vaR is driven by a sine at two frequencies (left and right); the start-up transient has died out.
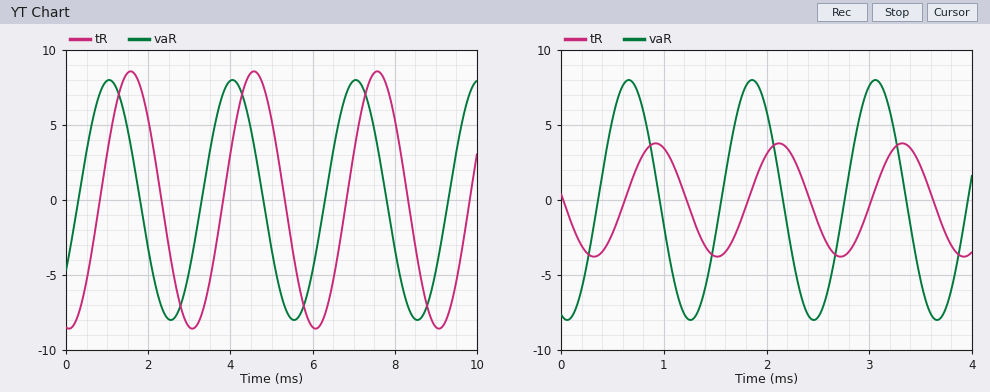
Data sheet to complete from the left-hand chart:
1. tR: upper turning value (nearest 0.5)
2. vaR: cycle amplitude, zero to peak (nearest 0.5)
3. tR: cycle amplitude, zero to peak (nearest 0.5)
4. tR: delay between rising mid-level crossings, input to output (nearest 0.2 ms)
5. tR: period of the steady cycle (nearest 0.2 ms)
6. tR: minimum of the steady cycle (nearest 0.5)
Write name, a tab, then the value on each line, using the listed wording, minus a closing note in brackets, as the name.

tR: upper turning value	8.5
vaR: cycle amplitude, zero to peak	8.0
tR: cycle amplitude, zero to peak	8.5
tR: delay between rising mid-level crossings, input to output	0.6 ms
tR: period of the steady cycle	3.0 ms
tR: minimum of the steady cycle	-8.5
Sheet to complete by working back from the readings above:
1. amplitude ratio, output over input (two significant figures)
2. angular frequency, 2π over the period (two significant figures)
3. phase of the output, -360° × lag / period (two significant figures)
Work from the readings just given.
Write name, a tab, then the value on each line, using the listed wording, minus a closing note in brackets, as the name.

amplitude ratio, output over input	1.1
angular frequency, 2π over the period	2.1 rad/ms
phase of the output, -360° × lag / period	-72°
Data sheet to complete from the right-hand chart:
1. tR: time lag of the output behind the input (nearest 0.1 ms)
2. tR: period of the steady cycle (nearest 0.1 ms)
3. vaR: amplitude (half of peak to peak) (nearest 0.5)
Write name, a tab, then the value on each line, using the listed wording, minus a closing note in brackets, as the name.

tR: time lag of the output behind the input	0.3 ms
tR: period of the steady cycle	1.2 ms
vaR: amplitude (half of peak to peak)	8.0
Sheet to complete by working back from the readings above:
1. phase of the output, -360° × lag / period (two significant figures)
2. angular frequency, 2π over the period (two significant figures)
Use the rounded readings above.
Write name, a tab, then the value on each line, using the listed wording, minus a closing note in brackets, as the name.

phase of the output, -360° × lag / period	-90°
angular frequency, 2π over the period	5.2 rad/ms
